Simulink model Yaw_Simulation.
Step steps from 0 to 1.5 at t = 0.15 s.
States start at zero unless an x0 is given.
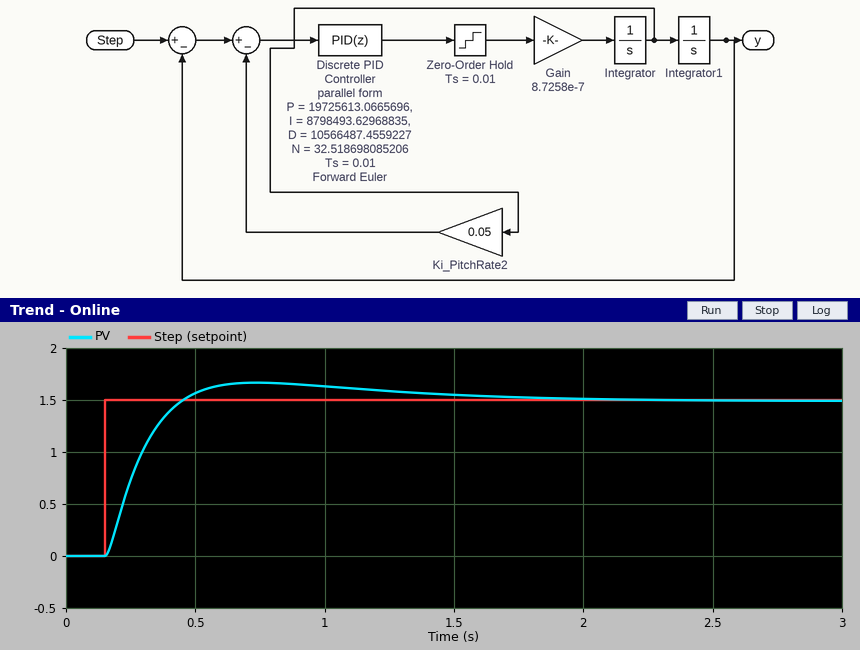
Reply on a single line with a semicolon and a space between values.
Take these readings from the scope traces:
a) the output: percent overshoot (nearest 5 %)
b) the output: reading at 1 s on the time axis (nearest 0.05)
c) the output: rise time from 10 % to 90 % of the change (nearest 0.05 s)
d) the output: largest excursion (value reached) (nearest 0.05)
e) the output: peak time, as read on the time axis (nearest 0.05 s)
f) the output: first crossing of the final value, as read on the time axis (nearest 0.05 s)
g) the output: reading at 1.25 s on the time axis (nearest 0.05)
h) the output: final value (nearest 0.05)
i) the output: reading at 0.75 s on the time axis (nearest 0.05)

10 %; 1.65; 0.20 s; 1.65; 0.75 s; 0.45 s; 1.60; 1.50; 1.65
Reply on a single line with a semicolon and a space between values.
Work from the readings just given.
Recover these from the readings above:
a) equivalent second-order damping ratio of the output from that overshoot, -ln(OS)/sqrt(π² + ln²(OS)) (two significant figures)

0.59
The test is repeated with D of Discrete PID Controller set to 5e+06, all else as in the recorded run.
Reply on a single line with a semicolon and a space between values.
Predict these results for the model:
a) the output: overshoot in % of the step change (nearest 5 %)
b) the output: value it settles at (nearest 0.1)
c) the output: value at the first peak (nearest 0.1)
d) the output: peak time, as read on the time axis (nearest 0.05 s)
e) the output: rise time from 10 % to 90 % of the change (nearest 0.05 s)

25 %; 1.5; 1.9; 0.80 s; 0.25 s
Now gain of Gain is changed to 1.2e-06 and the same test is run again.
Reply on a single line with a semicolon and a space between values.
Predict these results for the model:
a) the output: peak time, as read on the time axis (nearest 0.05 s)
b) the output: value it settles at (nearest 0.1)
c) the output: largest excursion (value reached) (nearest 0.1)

0.65 s; 1.5; 1.6
